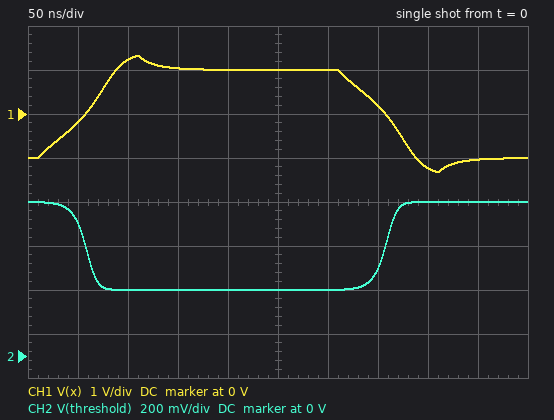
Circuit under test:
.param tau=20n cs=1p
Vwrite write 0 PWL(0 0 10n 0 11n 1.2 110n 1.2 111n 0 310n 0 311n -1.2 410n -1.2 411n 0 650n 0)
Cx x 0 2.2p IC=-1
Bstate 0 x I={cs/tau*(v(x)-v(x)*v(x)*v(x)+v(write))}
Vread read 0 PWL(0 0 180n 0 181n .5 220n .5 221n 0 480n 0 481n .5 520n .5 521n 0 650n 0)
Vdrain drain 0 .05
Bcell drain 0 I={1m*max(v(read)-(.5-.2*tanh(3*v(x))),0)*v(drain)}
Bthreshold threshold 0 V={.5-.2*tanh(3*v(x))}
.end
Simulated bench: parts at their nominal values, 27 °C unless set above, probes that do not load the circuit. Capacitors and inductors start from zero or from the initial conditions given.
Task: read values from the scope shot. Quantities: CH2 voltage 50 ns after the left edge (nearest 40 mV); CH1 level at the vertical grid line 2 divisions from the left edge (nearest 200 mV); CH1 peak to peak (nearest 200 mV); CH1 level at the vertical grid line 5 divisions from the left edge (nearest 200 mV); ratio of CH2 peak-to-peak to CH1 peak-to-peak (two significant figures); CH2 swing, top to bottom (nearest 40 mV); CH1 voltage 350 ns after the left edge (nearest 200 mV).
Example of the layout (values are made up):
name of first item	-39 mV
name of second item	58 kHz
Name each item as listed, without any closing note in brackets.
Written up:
CH2 voltage 50 ns after the left edge	600 mV
CH1 level at the vertical grid line 2 divisions from the left edge	1.2 V
CH1 peak to peak	2.6 V
CH1 level at the vertical grid line 5 divisions from the left edge	1.0 V
ratio of CH2 peak-to-peak to CH1 peak-to-peak	0.15
CH2 swing, top to bottom	400 mV
CH1 voltage 350 ns after the left edge	200 mV
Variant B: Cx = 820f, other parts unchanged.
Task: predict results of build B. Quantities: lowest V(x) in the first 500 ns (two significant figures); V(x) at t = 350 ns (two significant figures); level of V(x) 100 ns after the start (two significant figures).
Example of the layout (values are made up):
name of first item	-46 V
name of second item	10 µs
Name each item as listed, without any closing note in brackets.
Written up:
lowest V(x) in the first 500 ns	-1.4 V
V(x) at t = 350 ns	-1.3 V
level of V(x) 100 ns after the start	1.4 V
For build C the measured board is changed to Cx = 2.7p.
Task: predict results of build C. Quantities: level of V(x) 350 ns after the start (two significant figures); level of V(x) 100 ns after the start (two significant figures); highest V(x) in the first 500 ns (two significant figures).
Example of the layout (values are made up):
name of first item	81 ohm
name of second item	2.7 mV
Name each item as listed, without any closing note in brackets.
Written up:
level of V(x) 350 ns after the start	350 mV
level of V(x) 100 ns after the start	860 mV
highest V(x) in the first 500 ns	1.1 V
